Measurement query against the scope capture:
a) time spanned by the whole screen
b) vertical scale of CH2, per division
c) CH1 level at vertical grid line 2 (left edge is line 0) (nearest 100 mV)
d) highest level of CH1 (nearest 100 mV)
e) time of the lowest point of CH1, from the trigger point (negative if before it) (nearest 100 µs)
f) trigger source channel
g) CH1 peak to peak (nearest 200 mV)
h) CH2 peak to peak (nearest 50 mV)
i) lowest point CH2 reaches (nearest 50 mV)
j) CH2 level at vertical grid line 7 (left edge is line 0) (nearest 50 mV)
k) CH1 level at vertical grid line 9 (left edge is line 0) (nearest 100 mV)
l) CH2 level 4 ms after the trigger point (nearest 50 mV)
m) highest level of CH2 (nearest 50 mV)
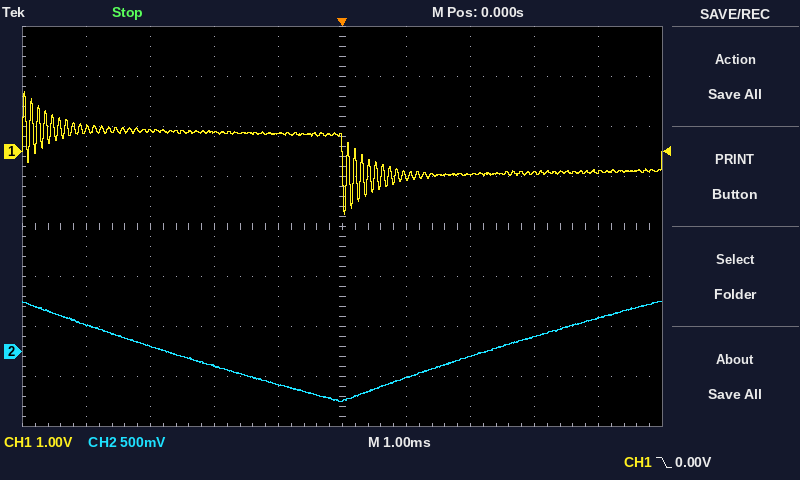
10 ms
500 mV
400 mV
1.2 V
0.0 ms
CH1
2.4 V
1.00 V
-500 mV
-50 mV
-400 mV
350 mV
500 mV
